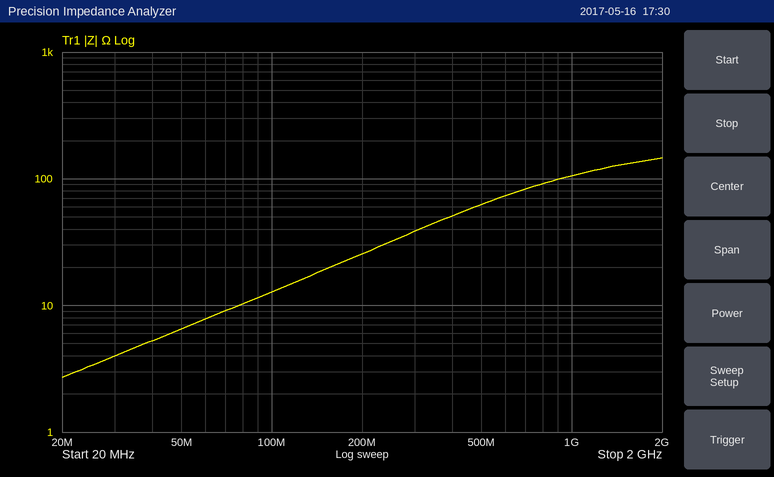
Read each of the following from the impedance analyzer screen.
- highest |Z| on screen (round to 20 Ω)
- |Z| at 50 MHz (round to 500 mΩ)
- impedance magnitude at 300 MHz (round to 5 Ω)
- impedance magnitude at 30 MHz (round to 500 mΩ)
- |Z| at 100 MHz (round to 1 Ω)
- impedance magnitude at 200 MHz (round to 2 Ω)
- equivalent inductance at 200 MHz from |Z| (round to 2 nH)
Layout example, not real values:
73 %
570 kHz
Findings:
140 Ω
6.5 Ω
40 Ω
4.0 Ω
13 Ω
26 Ω
20 nH
